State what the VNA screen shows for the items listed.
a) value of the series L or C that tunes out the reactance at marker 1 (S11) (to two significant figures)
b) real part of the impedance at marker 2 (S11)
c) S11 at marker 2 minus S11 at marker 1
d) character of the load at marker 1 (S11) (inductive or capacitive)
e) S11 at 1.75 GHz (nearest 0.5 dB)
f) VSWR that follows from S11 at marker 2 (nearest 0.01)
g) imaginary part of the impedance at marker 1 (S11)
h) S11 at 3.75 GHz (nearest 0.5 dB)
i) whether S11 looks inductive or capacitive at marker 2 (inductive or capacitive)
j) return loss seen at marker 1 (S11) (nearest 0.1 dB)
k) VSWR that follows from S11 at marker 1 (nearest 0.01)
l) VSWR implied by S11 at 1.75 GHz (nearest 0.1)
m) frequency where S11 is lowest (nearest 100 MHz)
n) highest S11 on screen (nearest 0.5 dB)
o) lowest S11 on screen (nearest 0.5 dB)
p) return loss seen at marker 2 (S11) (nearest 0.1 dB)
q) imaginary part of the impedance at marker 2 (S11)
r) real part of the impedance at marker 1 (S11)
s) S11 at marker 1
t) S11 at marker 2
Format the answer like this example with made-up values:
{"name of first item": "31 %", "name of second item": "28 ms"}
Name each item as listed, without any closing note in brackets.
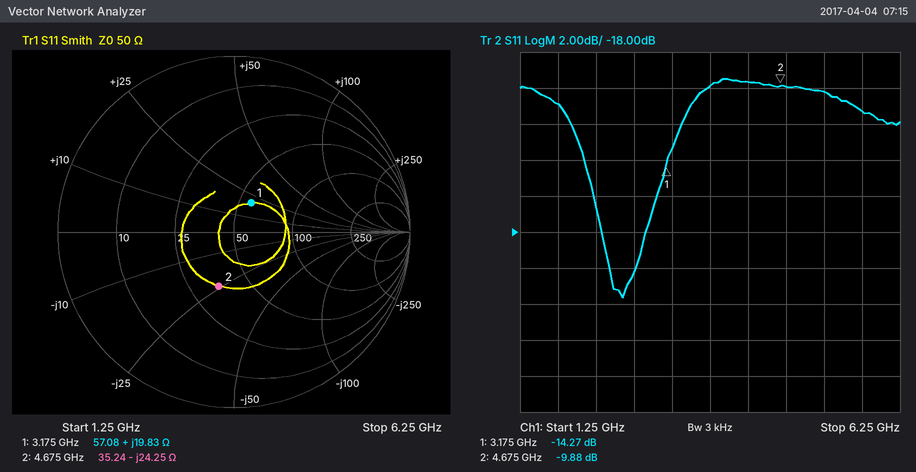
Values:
{"value of the series L or C that tunes out the reactance at marker 1 (S11)": "2.5 pF", "real part of the impedance at marker 2": "35.24 Ω", "S11 at marker 2 minus S11 at marker 1": "4.39 dB", "character of the load at marker 1 (S11)": "inductive", "S11 at 1.75 GHz": "-11.0 dB", "VSWR that follows from S11 at marker 2": "1.94", "imaginary part of the impedance at marker 1": "+19.83 Ω", "S11 at 3.75 GHz": "-10.0 dB", "whether S11 looks inductive or capacitive at marker 2": "capacitive", "return loss seen at marker 1 (S11)": "14.3 dB", "VSWR that follows from S11 at marker 1": "1.48", "VSWR implied by S11 at 1.75 GHz": "1.8", "frequency where S11 is lowest": "2.6 GHz", "highest S11 on screen": "-9.5 dB", "lowest S11 on screen": "-21.5 dB", "return loss seen at marker 2 (S11)": "9.9 dB", "imaginary part of the impedance at marker 2": "-24.25 Ω", "real part of the impedance at marker 1": "57.08 Ω", "S11 at marker 1": "-14.27 dB", "S11 at marker 2": "-9.88 dB"}
